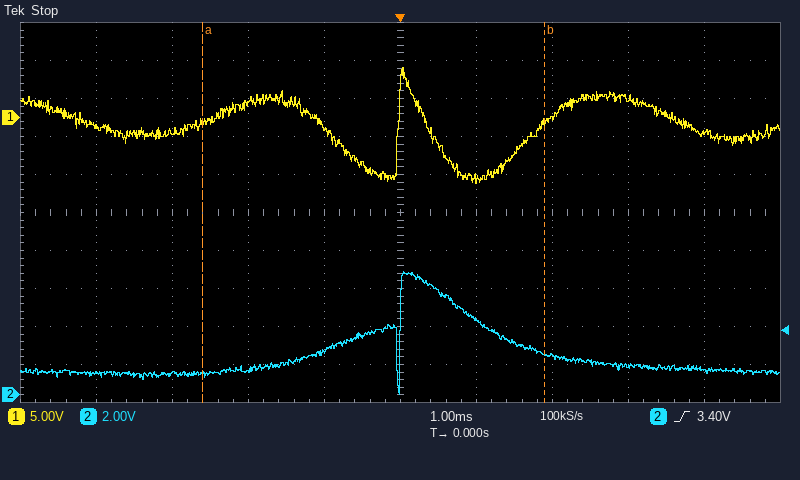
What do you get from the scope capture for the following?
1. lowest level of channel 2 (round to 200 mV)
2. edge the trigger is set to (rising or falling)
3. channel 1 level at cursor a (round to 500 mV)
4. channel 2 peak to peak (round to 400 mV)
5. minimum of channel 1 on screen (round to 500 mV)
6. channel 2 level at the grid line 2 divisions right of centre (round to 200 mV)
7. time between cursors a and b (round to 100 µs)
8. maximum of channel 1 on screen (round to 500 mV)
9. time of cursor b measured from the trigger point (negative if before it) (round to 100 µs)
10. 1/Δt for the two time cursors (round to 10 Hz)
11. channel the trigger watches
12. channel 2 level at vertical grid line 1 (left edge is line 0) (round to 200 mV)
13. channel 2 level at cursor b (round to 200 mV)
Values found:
0.0 V
rising
-500 mV
6.4 V
-8.5 V
2.0 V
4.5 ms
6.5 V
+1.9 ms
220 Hz
channel 2
1.2 V
2.2 V
